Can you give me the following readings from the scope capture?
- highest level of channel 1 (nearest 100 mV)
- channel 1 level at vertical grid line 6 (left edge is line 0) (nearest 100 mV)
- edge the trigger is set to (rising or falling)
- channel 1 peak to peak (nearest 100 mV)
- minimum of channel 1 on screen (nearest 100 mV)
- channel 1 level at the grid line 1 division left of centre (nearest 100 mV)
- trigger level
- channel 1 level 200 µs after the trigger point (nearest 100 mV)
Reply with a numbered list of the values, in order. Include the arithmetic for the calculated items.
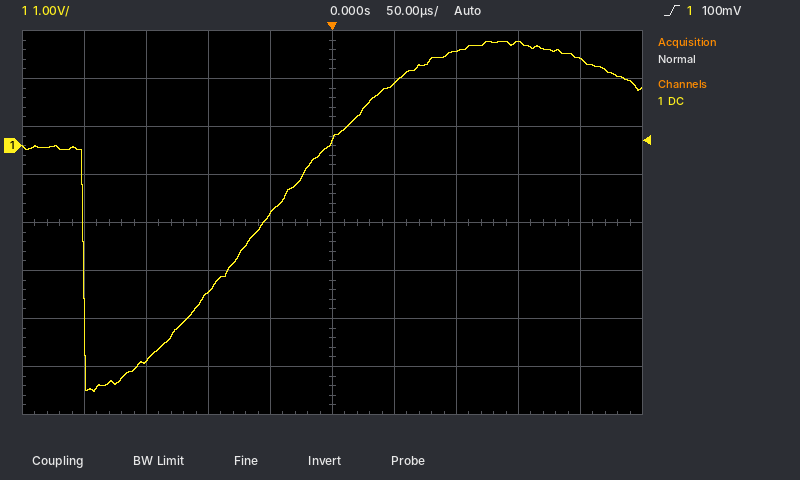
1. 2.2 V
2. 1.3 V
3. rising
4. 2.2 V − (-5.1 V) = 7.3 V
5. -5.1 V
6. -1.4 V
7. 100 mV
8. 1.8 V
